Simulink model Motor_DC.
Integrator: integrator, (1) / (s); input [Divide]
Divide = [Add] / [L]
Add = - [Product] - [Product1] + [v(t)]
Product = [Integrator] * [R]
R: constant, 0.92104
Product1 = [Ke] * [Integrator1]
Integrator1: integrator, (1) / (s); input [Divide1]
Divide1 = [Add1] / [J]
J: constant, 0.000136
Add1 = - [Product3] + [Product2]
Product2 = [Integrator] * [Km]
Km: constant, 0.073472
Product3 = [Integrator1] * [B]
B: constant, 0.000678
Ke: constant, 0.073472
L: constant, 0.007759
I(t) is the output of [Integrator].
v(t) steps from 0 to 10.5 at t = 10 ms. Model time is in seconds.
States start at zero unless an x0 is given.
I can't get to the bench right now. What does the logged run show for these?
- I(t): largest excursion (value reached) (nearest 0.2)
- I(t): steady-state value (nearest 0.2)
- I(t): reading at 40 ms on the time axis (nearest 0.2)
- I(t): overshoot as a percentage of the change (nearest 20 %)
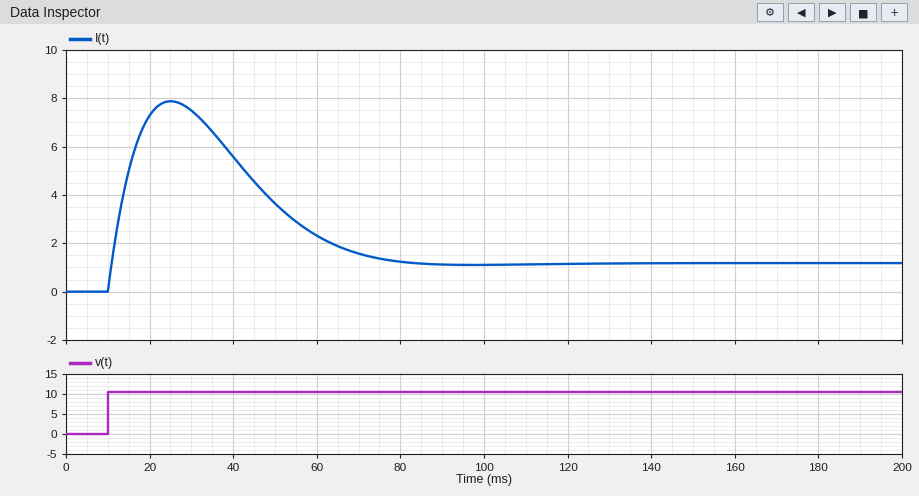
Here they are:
7.8
1.2
5.6
560 %
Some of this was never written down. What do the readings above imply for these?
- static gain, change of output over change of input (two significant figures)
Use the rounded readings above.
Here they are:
0.11
